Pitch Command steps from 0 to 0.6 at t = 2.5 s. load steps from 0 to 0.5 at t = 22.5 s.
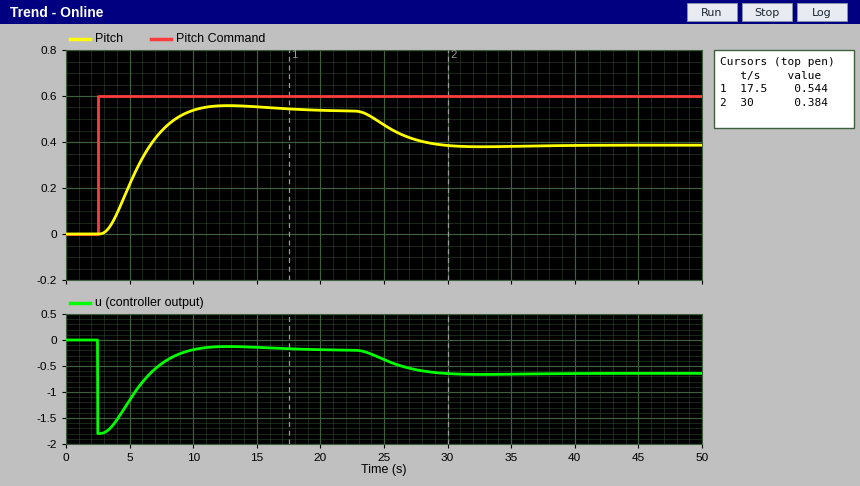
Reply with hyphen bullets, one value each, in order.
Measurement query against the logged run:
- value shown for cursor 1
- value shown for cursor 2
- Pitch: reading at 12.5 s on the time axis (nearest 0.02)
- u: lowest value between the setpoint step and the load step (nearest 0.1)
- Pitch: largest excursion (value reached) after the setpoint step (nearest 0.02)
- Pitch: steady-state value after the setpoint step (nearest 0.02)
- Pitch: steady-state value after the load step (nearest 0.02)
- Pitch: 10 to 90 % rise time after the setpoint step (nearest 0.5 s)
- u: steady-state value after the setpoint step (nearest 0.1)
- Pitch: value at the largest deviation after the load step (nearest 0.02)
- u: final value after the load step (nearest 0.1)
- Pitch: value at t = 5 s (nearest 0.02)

- 0.544
- 0.384
- 0.56
- -1.8
- 0.56
- 0.54
- 0.38
- 4.5 s
- -0.2
- 0.38
- -0.6
- 0.22
